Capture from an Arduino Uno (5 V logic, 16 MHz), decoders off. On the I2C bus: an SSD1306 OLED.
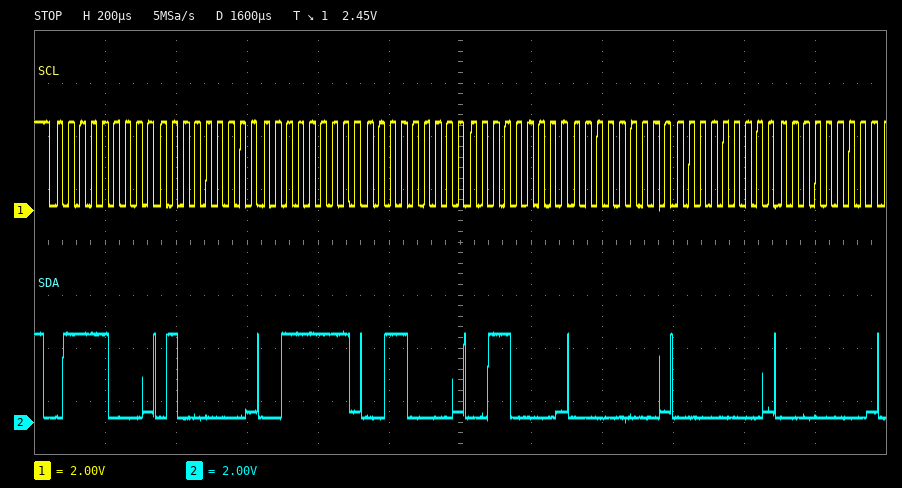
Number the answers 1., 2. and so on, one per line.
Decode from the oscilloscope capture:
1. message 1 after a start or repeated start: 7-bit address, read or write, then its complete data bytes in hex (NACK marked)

1. 0x3C write: 40 3F 30 30 00 00 00
